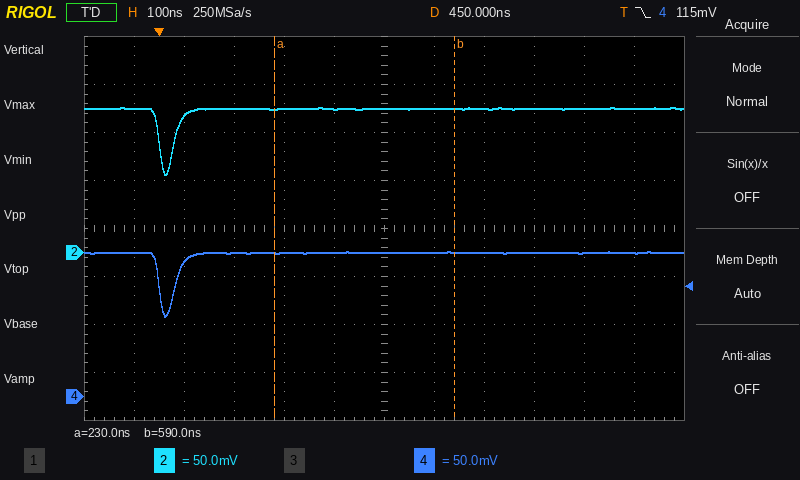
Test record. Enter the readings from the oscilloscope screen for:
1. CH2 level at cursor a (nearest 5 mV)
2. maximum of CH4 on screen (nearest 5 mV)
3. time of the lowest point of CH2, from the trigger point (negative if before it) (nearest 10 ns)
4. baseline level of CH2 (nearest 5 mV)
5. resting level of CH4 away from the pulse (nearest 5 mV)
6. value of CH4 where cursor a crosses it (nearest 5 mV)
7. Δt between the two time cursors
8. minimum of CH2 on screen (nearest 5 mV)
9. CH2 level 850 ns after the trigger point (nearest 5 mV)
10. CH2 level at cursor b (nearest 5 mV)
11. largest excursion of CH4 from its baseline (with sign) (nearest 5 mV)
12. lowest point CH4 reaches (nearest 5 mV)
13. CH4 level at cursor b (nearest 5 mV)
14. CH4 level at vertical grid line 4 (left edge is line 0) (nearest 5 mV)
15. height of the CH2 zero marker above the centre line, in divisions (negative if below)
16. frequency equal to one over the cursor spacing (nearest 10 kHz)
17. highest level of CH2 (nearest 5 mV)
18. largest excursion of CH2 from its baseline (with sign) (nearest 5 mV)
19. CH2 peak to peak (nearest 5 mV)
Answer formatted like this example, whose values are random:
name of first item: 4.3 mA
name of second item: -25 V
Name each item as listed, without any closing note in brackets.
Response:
CH2 level at cursor a: 150 mV
maximum of CH4 on screen: 150 mV
time of the lowest point of CH2, from the trigger point (negative if before it): +10 ns
baseline level of CH2: 150 mV
resting level of CH4 away from the pulse: 150 mV
value of CH4 where cursor a crosses it: 150 mV
Δt between the two time cursors: 360 ns
minimum of CH2 on screen: 80 mV
CH2 level 850 ns after the trigger point: 150 mV
CH2 level at cursor b: 150 mV
largest excursion of CH4 from its baseline (with sign): -65 mV
lowest point CH4 reaches: 85 mV
CH4 level at cursor b: 150 mV
CH4 level at vertical grid line 4 (left edge is line 0): 150 mV
height of the CH2 zero marker above the centre line, in divisions: -0.5 div
frequency equal to one over the cursor spacing: 2.78 MHz
highest level of CH2: 150 mV
largest excursion of CH2 from its baseline (with sign): -70 mV
CH2 peak to peak: 70 mV
